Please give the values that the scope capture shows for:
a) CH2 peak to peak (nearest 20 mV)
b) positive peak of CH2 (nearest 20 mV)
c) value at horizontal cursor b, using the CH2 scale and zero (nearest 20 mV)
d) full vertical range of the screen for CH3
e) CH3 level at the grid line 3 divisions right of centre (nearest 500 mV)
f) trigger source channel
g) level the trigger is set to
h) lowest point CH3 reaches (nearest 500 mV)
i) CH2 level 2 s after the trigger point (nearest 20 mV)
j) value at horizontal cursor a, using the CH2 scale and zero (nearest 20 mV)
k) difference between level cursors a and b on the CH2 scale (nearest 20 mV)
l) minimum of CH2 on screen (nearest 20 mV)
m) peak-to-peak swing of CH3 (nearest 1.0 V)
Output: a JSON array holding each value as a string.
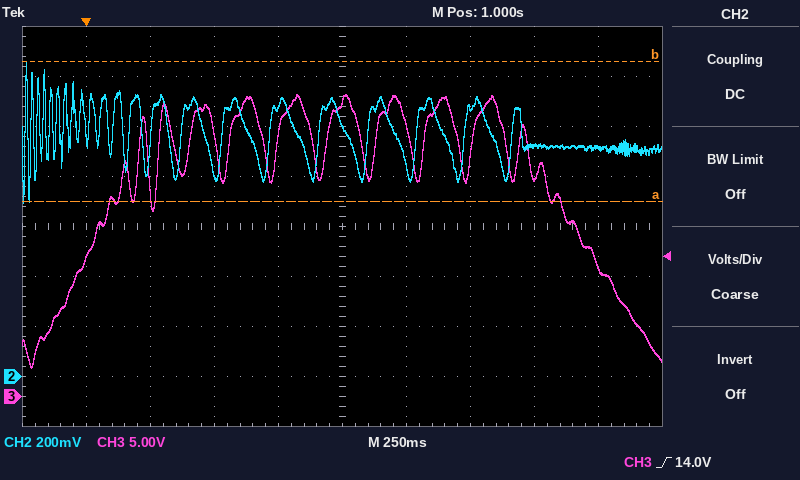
["560 mV", "1.26 V", "1.26 V", "40 V", "22.0 V", "CH3", "14.0 V", "3.0 V", "920 mV", "700 mV", "560 mV", "700 mV", "27.0 V"]
